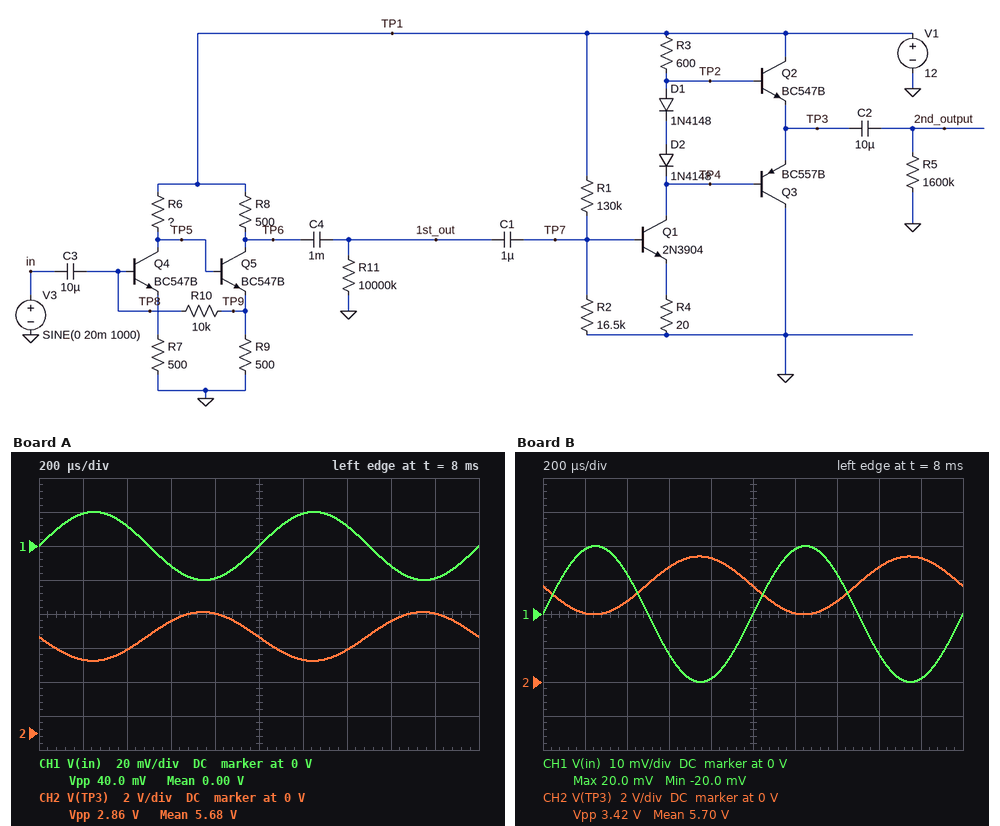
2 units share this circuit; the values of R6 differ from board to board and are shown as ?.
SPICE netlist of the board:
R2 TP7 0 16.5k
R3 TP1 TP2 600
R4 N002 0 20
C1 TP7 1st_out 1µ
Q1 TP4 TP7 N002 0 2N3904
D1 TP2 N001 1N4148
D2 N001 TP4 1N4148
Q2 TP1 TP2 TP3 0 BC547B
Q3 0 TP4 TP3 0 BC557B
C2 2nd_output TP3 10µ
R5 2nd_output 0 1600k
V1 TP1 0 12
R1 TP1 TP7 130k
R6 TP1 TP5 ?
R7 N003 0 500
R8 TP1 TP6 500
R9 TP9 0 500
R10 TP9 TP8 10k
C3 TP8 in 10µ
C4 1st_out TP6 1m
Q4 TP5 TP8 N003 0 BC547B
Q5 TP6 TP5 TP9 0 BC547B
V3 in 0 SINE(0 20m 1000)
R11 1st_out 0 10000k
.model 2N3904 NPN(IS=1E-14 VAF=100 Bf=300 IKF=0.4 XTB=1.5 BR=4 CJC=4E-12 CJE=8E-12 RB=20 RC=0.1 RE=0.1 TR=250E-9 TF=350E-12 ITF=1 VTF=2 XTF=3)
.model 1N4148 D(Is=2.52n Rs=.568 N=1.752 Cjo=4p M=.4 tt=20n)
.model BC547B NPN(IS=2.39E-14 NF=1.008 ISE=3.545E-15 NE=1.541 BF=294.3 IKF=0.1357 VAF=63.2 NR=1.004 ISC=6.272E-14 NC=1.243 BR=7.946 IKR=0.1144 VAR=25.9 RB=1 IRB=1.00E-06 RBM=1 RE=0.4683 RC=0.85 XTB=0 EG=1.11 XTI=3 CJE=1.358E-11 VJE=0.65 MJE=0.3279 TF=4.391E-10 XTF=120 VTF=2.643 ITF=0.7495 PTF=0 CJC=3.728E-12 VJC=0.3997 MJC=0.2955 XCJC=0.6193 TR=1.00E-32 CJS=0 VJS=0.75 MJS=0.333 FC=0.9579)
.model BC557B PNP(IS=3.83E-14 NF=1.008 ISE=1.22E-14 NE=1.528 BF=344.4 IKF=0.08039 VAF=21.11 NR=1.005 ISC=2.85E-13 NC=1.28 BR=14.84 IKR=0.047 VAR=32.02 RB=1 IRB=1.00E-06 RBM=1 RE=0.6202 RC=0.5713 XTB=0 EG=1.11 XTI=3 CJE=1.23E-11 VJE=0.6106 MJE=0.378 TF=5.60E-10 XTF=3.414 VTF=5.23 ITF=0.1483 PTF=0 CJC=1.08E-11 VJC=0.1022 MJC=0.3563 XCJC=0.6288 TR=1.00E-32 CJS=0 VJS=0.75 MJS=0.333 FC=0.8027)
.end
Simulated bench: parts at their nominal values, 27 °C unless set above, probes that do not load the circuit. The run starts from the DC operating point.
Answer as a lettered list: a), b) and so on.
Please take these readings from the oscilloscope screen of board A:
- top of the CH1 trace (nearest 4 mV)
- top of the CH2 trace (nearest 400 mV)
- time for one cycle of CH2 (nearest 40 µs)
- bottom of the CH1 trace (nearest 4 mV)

a) 20 mV
b) 7.2 V
c) 1.00 ms
d) -20 mV
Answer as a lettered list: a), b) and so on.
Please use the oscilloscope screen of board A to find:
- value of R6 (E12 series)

a) 1.5 kΩ
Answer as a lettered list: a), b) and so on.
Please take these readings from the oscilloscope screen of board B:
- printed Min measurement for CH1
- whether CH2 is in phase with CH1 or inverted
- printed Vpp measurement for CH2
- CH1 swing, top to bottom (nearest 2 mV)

a) -20.0 mV
b) inverted
c) 3.42 V
d) 40 mV
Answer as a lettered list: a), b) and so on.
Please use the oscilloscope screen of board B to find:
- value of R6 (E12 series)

a) 1.8 kΩ
